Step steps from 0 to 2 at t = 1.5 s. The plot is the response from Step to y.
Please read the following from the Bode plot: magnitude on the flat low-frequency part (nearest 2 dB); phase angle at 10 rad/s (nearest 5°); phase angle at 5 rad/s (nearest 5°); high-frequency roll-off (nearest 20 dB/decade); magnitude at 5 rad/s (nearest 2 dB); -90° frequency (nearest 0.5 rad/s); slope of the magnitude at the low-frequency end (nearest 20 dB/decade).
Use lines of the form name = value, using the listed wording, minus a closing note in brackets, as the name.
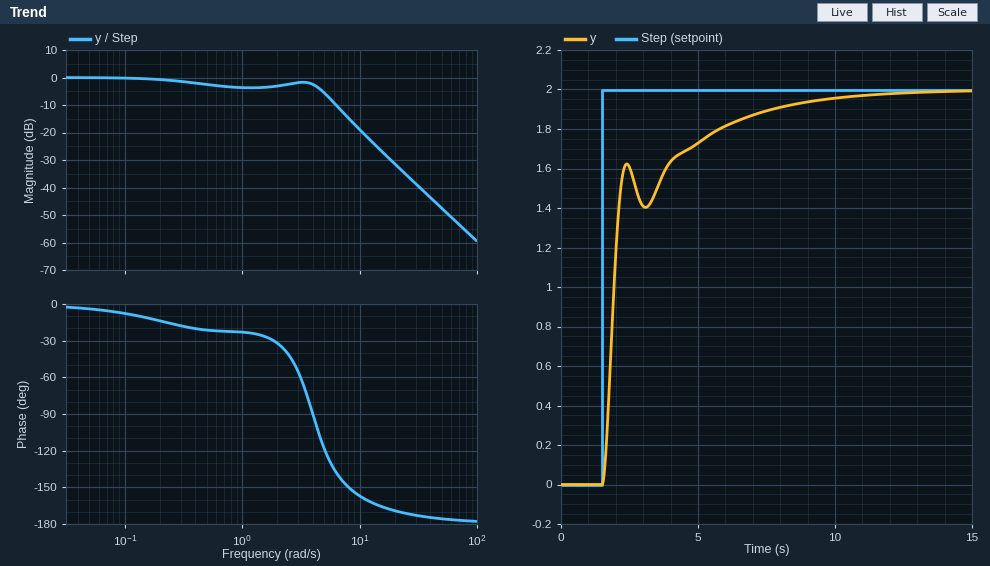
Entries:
magnitude on the flat low-frequency part = 0 dB
phase angle at 10 rad/s = -155°
phase angle at 5 rad/s = -120°
high-frequency roll-off = -40 dB/decade
magnitude at 5 rad/s = -6 dB
-90° frequency = 4.0 rad/s
slope of the magnitude at the low-frequency end = 0 dB/decade
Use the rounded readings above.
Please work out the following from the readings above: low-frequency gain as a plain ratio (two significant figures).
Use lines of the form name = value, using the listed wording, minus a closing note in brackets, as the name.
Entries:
low-frequency gain as a plain ratio = 1.0
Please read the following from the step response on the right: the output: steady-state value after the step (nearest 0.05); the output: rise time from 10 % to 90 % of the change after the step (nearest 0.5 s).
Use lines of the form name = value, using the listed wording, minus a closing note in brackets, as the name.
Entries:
the output: steady-state value after the step = 2.00
the output: rise time from 10 % to 90 % of the change after the step = 4.0 s
